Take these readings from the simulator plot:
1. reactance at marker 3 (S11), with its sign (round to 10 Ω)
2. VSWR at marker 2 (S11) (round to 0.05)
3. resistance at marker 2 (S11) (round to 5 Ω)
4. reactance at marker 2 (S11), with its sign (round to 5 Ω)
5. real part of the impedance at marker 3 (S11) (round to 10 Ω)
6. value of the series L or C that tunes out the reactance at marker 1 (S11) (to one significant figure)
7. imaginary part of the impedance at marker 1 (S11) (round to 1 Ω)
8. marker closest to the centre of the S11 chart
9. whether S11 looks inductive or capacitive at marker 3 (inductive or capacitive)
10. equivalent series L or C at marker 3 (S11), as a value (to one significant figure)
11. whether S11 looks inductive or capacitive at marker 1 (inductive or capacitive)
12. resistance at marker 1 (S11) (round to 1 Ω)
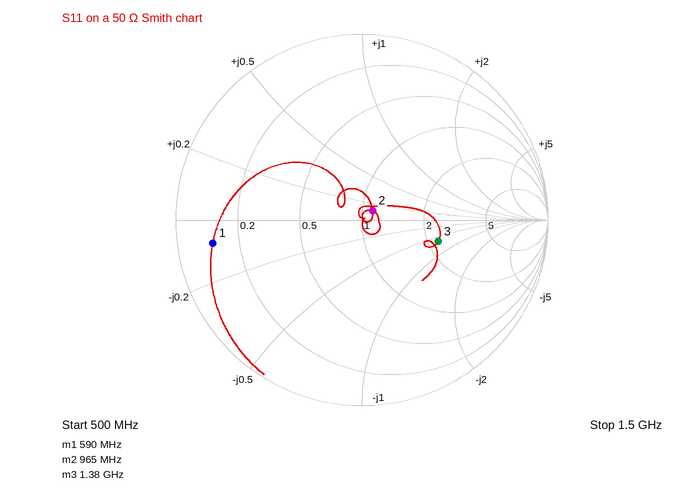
-30 Ω
1.15
55 Ω
+5 Ω
110 Ω
1 nH
-4 Ω
marker 2
capacitive
4 pF
capacitive
5 Ω
